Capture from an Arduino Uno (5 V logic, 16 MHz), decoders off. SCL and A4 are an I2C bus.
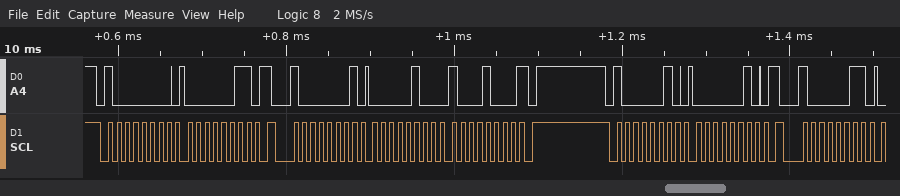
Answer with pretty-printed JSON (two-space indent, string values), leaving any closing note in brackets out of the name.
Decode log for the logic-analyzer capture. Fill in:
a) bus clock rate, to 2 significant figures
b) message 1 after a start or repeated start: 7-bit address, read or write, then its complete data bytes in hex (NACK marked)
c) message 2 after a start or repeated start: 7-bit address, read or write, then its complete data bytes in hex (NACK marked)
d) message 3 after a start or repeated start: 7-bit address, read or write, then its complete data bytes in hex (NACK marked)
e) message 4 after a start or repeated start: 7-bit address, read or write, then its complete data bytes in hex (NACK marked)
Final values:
{
  "bus clock rate, to 2 significant figures": "100 kHz",
  "message 1 after a start or repeated start: 7-bit address, read or write, then its complete data bytes in hex": "0x40 write: 03",
  "message 2 after a start or repeated start: 7-bit address, read or write, then its complete data bytes in hex": "0x40 read: 04 88 NACK",
  "message 3 after a start or repeated start: 7-bit address, read or write, then its complete data bytes in hex": "0x41 write: 02",
  "message 4 after a start or repeated start: 7-bit address, read or write, then its complete data bytes in hex": "0x41 read"
}
